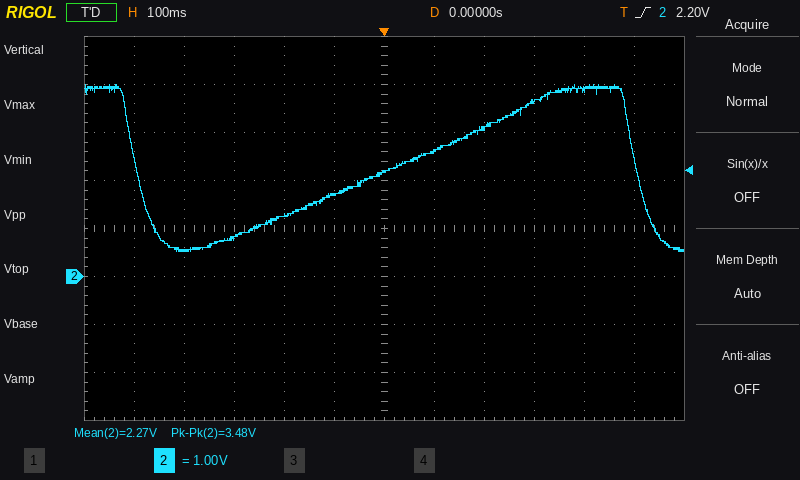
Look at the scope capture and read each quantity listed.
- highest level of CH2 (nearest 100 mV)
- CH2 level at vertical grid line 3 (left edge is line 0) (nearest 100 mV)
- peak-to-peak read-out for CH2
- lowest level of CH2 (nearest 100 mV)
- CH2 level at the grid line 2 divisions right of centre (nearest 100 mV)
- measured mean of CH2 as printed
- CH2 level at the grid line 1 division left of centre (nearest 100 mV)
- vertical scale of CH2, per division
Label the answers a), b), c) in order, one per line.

a) 4.0 V
b) 800 mV
c) 3.48 V
d) 500 mV
e) 3.1 V
f) 2.27 V
g) 1.7 V
h) 1 V
